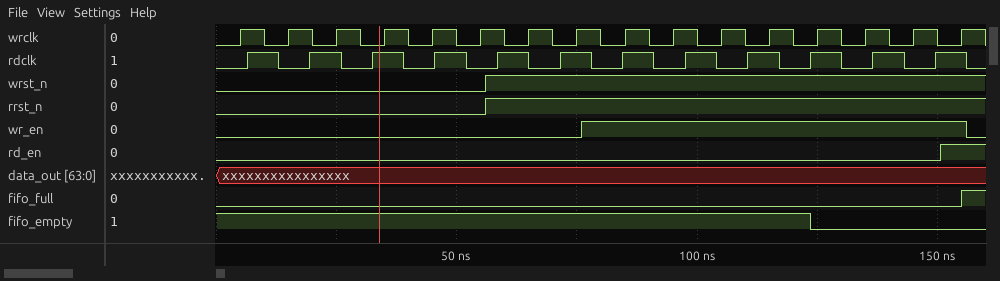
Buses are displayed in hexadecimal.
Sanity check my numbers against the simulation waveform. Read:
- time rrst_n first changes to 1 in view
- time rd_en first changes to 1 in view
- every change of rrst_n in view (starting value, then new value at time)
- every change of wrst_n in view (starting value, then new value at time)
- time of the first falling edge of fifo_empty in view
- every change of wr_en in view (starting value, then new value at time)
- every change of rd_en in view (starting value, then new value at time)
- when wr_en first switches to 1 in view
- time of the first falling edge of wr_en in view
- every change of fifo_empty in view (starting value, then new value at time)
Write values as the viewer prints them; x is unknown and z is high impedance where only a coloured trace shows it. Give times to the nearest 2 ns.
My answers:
56 ns
150 ns
0, 1 at 56 ns
0, 1 at 56 ns
124 ns
0, 1 at 76 ns, 0 at 156 ns
0, 1 at 150 ns
76 ns
156 ns
1, 0 at 124 ns
